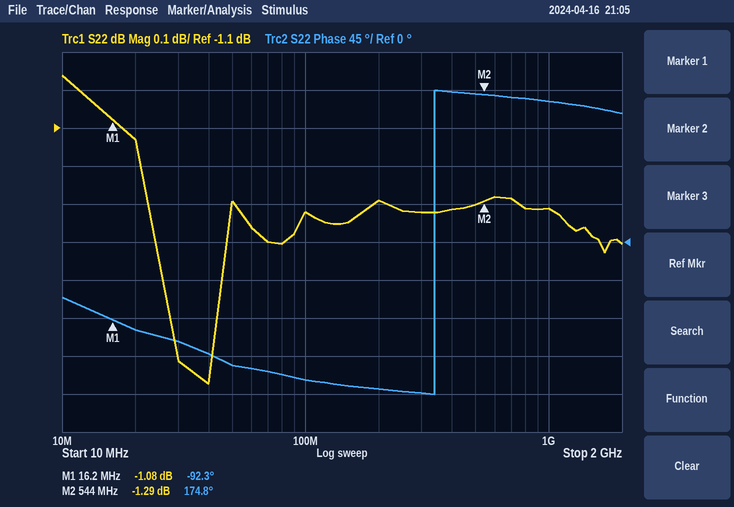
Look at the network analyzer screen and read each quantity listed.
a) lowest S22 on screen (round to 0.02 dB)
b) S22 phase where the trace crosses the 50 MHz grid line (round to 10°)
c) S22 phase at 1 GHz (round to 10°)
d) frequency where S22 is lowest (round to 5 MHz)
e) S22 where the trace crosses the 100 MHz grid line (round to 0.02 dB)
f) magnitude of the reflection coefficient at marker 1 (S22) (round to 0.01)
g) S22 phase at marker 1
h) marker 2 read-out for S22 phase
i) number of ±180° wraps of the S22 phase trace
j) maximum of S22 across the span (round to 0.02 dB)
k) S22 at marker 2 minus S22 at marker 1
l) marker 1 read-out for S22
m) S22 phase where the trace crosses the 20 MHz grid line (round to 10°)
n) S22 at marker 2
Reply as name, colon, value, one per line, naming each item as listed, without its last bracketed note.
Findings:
lowest S22 on screen: -1.78 dB
S22 phase where the trace crosses the 50 MHz grid line: -150°
S22 phase at 1 GHz: 170°
frequency where S22 is lowest: 40 MHz
S22 where the trace crosses the 100 MHz grid line: -1.32 dB
magnitude of the reflection coefficient at marker 1 (S22): 0.88
S22 phase at marker 1: -92.3°
marker 2 read-out for S22 phase: 174.8°
number of ±180° wraps of the S22 phase trace: 1
maximum of S22 across the span: -0.96 dB
S22 at marker 2 minus S22 at marker 1: -0.21 dB
marker 1 read-out for S22: -1.08 dB
S22 phase where the trace crosses the 20 MHz grid line: -100°
S22 at marker 2: -1.29 dB
